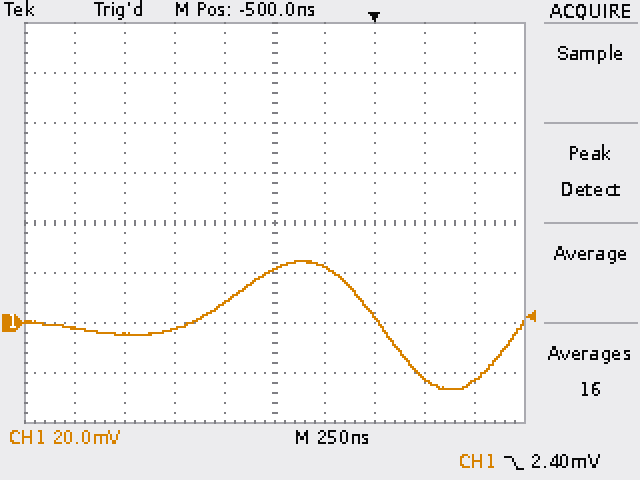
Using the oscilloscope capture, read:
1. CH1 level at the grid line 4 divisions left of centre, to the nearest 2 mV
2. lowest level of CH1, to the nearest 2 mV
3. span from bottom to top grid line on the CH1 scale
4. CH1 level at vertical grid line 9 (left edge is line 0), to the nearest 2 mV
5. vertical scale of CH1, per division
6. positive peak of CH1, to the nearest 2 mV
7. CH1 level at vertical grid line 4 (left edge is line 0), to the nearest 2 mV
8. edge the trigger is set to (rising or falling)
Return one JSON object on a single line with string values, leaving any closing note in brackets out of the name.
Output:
{"CH1 level at the grid line 4 divisions left of centre, to the nearest 2 mV": "-2 mV", "lowest level of CH1, to the nearest 2 mV": "-26 mV", "span from bottom to top grid line on the CH1 scale": "160 mV", "CH1 level at vertical grid line 9 (left edge is line 0), to the nearest 2 mV": "-24 mV", "vertical scale of CH1, per division": "20 mV", "positive peak of CH1, to the nearest 2 mV": "24 mV", "CH1 level at vertical grid line 4 (left edge is line 0), to the nearest 2 mV": "8 mV", "edge the trigger is set to": "falling"}
